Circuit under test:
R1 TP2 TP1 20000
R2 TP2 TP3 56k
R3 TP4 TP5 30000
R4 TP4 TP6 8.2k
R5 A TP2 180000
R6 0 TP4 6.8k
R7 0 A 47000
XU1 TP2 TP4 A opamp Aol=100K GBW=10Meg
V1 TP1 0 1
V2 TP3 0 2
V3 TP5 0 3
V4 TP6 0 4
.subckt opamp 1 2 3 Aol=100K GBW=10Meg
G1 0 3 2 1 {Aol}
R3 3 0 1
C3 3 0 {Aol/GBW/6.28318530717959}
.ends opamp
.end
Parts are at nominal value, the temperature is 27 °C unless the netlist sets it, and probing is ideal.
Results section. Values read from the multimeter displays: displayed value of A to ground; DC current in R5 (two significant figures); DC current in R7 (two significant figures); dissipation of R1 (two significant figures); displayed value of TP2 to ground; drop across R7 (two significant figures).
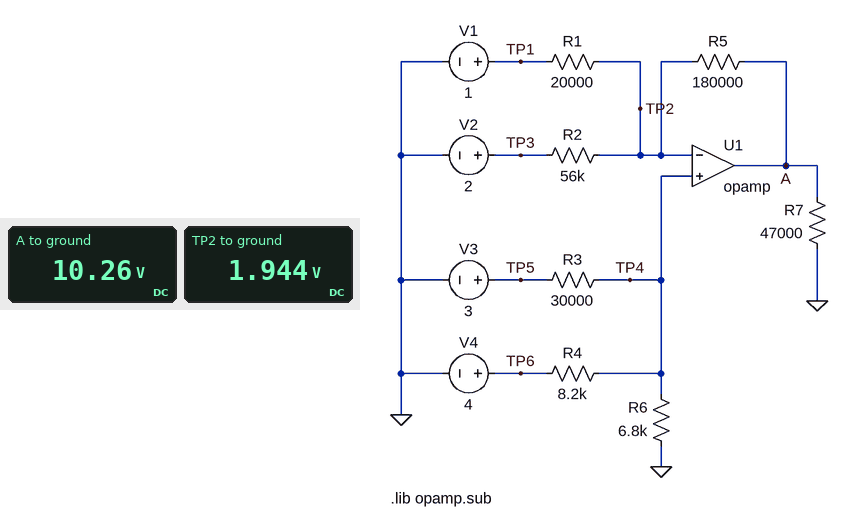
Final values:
10.26 V
46 µA
220 µA
45 µW
1.944 V
10 V
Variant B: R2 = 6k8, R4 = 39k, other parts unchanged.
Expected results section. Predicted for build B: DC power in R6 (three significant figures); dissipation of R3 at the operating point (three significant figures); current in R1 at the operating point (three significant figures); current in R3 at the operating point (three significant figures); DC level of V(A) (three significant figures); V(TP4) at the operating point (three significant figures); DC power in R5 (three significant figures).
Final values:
142 µW
136 µW
829 nA
67.2 µA
-26.1 V
983 mV
4.07 mW
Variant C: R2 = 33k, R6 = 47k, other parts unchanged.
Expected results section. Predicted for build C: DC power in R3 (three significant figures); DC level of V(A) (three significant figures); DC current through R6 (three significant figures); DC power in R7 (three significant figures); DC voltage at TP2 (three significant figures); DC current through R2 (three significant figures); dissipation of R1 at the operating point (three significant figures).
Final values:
3.61 µW
31.5 V
70.8 µA
21.2 mW
3.33 V
40.3 µA
271 µW
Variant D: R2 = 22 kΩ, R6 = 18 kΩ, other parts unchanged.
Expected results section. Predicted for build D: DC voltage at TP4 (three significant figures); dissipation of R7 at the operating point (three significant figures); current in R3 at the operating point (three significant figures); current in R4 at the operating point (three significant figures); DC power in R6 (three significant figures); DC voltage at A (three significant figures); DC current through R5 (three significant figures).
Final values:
2.79 V
13.6 mW
7.07 µA
148 µA
432 µW
25.3 V
125 µA
